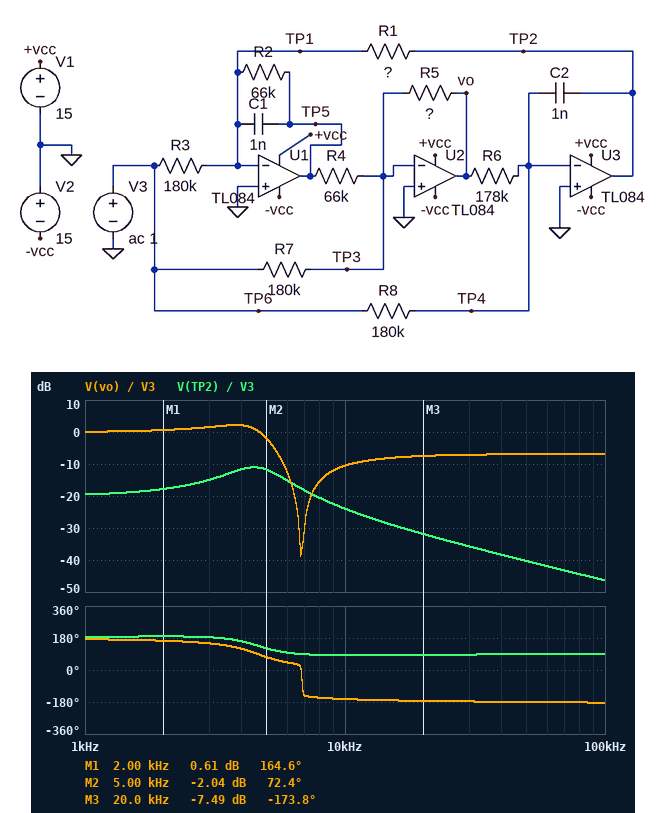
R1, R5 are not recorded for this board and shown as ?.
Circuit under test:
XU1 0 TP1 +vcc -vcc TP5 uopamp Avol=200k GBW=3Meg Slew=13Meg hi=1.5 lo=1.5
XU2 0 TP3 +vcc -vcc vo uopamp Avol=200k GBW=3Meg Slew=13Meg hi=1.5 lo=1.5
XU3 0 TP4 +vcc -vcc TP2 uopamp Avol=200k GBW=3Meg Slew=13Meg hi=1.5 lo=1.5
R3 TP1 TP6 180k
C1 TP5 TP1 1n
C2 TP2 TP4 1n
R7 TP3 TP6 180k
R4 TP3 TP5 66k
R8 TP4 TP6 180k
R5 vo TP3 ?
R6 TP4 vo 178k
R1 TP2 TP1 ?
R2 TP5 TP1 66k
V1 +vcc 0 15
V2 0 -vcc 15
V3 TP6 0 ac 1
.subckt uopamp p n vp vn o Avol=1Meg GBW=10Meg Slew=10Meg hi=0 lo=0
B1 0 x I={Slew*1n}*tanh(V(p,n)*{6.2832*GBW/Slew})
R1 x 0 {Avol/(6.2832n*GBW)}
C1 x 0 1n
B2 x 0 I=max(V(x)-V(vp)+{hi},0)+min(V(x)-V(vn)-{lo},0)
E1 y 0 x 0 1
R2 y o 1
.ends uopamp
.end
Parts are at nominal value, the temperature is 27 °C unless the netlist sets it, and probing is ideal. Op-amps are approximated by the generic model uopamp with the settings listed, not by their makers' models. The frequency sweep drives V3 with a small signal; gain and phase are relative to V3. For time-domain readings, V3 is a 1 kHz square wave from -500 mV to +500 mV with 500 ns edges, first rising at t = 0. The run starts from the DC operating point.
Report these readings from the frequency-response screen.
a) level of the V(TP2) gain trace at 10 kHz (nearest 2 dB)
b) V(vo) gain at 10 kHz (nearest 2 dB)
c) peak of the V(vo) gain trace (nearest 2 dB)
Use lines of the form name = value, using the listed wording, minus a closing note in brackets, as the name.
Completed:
level of the V(TP2) gain trace at 10 kHz = -24 dB
V(vo) gain at 10 kHz = -10 dB
peak of the V(vo) gain trace = 2 dB
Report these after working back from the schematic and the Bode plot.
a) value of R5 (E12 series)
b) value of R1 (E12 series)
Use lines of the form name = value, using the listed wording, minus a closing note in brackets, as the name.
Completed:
value of R5 = 82 kΩ
value of R1 = 8.2 kΩ
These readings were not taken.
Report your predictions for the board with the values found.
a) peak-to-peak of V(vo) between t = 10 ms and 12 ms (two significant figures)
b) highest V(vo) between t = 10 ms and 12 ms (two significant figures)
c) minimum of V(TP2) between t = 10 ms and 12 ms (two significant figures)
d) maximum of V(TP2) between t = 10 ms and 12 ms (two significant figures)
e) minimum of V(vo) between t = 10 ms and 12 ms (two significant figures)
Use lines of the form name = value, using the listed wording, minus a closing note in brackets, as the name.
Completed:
peak-to-peak of V(vo) between t = 10 ms and 12 ms = 1.5 V
highest V(vo) between t = 10 ms and 12 ms = 740 mV
minimum of V(TP2) between t = 10 ms and 12 ms = -120 mV
maximum of V(TP2) between t = 10 ms and 12 ms = 120 mV
minimum of V(vo) between t = 10 ms and 12 ms = -740 mV
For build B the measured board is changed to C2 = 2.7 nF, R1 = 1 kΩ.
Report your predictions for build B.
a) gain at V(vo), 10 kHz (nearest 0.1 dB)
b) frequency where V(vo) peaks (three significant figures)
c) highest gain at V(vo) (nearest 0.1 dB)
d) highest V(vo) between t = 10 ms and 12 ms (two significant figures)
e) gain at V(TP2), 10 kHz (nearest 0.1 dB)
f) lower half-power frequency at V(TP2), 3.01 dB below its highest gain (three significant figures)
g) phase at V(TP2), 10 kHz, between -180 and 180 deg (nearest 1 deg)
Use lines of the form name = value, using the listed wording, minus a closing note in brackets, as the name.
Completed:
gain at V(vo), 10 kHz = -8.8 dB
frequency where V(vo) peaks = 7.47 kHz
highest gain at V(vo) = 6.2 dB
highest V(vo) between t = 10 ms and 12 ms = 840 mV
gain at V(TP2), 10 kHz = -27.2 dB
lower half-power frequency at V(TP2), 3.01 dB below its highest gain = 6.79 kHz
phase at V(TP2), 10 kHz, between -180 and 180 deg = 97 deg
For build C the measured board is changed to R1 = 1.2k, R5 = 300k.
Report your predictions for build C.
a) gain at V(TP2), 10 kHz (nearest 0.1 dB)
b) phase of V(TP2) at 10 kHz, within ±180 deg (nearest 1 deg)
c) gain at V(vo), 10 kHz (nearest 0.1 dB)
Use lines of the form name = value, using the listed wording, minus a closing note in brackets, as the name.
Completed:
gain at V(TP2), 10 kHz = -36.4 dB
phase of V(TP2) at 10 kHz, within ±180 deg = 104 deg
gain at V(vo), 10 kHz = -1.7 dB
